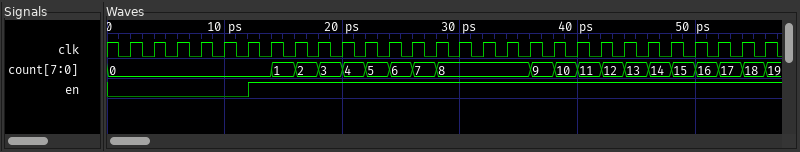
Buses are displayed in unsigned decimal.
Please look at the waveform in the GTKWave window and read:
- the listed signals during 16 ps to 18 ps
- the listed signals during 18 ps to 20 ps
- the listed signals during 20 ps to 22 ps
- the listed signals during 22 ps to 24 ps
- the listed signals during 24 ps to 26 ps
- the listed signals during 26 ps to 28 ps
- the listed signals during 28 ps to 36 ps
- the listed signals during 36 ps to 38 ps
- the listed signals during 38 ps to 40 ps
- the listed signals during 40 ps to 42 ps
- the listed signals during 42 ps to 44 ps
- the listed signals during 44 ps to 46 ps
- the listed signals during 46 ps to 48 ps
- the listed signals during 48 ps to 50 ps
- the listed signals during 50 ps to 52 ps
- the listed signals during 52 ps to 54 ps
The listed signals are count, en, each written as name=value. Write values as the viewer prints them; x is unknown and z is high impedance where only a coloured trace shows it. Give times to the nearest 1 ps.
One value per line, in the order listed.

count=2, en=1
count=3, en=1
count=4, en=1
count=5, en=1
count=6, en=1
count=7, en=1
count=8, en=1
count=9, en=1
count=10, en=1
count=11, en=1
count=12, en=1
count=13, en=1
count=14, en=1
count=15, en=1
count=16, en=1
count=17, en=1
